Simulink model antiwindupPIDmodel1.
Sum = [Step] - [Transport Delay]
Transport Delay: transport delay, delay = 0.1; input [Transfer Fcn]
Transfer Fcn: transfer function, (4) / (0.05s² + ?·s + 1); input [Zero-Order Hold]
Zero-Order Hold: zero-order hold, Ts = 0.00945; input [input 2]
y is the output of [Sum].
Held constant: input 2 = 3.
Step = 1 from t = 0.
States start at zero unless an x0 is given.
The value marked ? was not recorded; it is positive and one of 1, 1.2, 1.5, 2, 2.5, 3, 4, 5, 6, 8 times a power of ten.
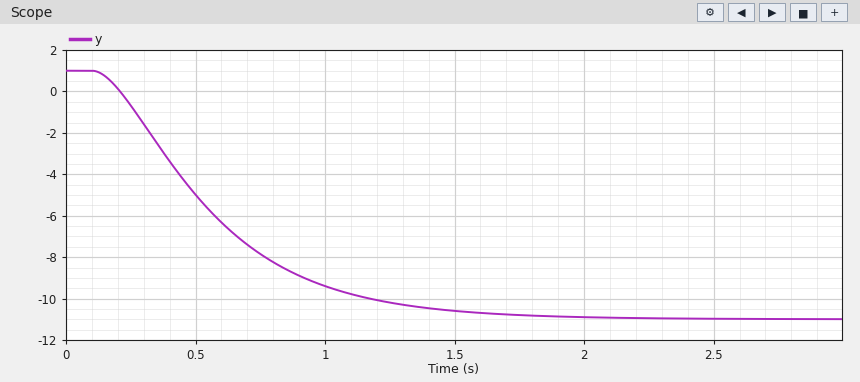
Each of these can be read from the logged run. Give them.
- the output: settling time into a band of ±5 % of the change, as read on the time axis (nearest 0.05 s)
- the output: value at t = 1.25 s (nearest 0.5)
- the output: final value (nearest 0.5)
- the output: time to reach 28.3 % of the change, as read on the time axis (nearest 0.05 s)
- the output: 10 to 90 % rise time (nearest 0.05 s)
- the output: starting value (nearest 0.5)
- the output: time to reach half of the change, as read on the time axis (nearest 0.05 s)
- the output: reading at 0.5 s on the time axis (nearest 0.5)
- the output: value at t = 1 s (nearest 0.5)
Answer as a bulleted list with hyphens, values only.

- 1.35 s
- -10.0
- -11.0
- 0.35 s
- 0.90 s
- 1.0
- 0.50 s
- -5.0
- -9.5
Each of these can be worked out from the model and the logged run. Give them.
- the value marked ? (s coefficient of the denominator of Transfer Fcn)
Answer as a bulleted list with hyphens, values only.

- 0.5
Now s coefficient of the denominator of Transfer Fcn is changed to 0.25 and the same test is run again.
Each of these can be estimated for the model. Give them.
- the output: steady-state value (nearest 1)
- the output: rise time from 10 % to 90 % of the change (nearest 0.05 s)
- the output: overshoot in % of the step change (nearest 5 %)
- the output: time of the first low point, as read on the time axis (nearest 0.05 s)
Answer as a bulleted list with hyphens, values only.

- -11
- 0.40 s
- 10 %
- 0.95 s
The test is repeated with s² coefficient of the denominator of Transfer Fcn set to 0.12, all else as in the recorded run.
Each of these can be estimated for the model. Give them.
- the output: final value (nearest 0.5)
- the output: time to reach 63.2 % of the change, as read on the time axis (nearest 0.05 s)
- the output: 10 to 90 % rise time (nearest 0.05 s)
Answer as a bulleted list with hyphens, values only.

- -11.0
- 0.70 s
- 0.75 s
